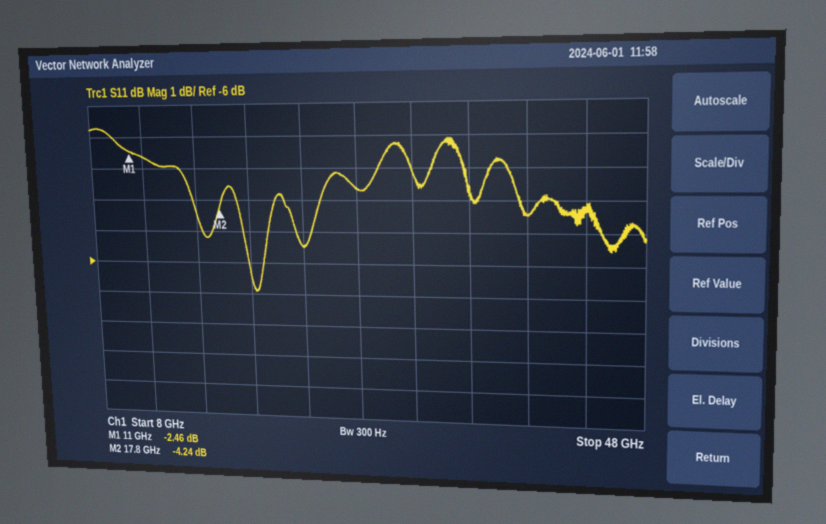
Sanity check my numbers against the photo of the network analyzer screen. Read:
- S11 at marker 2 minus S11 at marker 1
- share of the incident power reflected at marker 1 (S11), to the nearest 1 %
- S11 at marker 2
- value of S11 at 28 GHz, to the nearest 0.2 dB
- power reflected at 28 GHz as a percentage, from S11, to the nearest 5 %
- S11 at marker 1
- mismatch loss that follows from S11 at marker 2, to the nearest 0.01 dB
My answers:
-1.78 dB
57 %
-4.24 dB
-3.6 dB
45 %
-2.46 dB
2.05 dB
